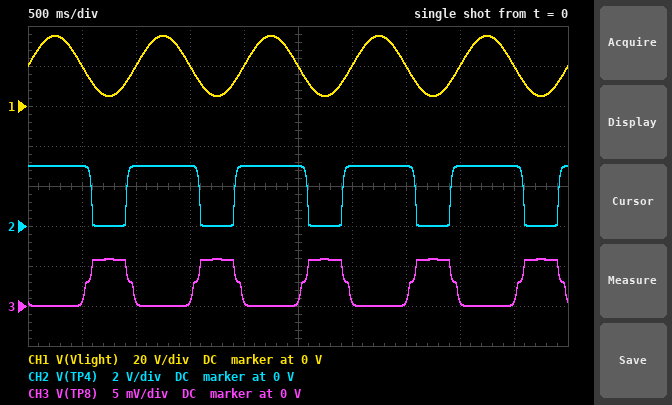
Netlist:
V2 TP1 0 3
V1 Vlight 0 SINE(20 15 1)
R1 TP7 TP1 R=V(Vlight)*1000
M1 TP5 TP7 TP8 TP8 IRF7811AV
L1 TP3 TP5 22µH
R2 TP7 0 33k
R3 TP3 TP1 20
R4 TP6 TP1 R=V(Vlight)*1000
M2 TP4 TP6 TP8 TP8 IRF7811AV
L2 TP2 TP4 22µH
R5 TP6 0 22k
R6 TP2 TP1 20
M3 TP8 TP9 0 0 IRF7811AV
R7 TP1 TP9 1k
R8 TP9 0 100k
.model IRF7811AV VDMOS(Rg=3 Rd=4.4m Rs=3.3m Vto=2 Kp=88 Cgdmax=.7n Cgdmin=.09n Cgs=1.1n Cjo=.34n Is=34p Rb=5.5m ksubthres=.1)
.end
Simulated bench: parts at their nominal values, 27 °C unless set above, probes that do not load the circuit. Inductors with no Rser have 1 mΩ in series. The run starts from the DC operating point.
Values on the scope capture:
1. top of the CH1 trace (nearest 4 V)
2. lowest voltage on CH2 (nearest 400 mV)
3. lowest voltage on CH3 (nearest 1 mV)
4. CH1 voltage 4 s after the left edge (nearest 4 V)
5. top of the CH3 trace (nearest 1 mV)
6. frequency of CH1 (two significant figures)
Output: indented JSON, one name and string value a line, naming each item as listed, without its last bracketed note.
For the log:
{
  "top of the CH1 trace": "36 V",
  "lowest voltage on CH2": "0 V",
  "lowest voltage on CH3": "0 V",
  "CH1 voltage 4 s after the left edge": "20 V",
  "top of the CH3 trace": "6 mV",
  "frequency of CH1": "1.0 Hz"
}
